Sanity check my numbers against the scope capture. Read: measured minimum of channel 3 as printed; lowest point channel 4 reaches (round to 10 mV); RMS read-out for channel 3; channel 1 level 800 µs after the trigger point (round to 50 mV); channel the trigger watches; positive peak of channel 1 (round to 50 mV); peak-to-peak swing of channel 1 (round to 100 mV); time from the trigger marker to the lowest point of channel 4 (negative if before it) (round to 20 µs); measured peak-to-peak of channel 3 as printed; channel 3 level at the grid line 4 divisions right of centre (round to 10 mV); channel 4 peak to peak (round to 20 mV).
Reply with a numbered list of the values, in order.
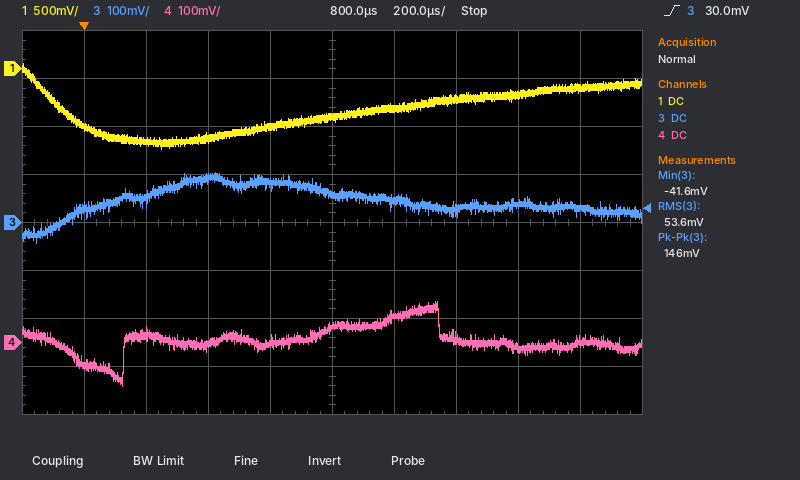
1. -41.6 mV
2. -90 mV
3. 53.6 mV
4. -500 mV
5. channel 3
6. 50 mV
7. 900 mV
8. +120 µs
9. 146 mV
10. 30 mV
11. 180 mV
